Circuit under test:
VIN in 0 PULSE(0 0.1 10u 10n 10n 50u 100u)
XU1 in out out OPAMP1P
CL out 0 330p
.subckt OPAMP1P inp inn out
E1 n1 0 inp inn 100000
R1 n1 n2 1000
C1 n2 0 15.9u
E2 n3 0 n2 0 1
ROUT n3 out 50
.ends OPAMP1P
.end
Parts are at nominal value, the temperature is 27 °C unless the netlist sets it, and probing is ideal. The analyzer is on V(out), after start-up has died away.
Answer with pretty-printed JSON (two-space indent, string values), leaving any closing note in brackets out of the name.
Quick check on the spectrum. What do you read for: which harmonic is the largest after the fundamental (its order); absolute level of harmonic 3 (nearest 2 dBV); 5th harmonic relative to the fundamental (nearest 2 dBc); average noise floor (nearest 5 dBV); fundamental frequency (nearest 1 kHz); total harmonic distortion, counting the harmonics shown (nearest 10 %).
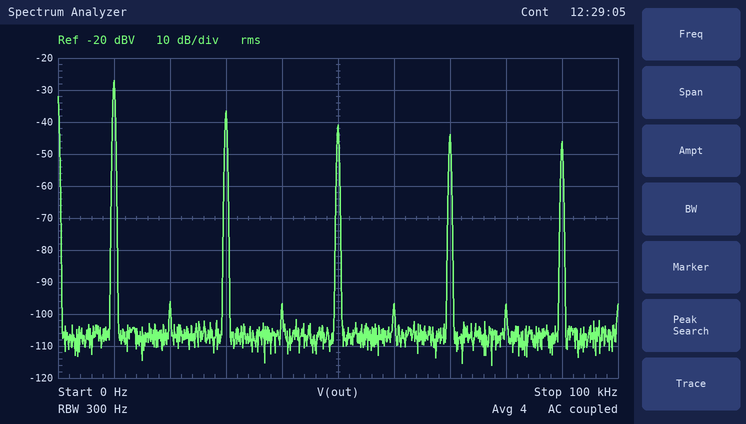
{
  "which harmonic is the largest after the fundamental": "3",
  "absolute level of harmonic 3": "-36 dBV",
  "5th harmonic relative to the fundamental": "-14 dBc",
  "average noise floor": "-105 dBV",
  "fundamental frequency": "10 kHz",
  "total harmonic distortion, counting the harmonics shown": "40 %"
}
